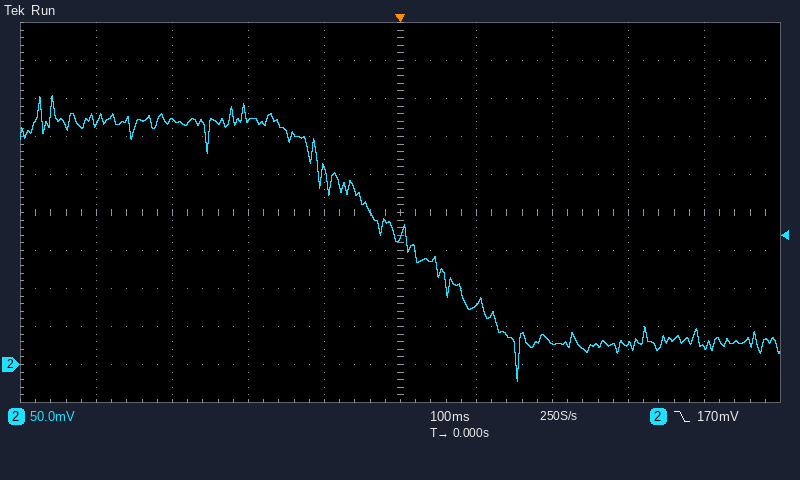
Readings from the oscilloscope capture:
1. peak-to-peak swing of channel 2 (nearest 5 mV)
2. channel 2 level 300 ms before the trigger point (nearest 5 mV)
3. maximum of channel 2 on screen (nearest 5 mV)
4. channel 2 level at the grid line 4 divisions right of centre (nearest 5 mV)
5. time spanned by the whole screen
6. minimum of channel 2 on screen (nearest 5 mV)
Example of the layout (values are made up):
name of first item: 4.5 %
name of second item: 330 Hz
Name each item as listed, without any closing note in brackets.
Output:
peak-to-peak swing of channel 2: 375 mV
channel 2 level 300 ms before the trigger point: 320 mV
maximum of channel 2 on screen: 355 mV
channel 2 level at the grid line 4 divisions right of centre: 25 mV
time spanned by the whole screen: 1 s
minimum of channel 2 on screen: -20 mV
